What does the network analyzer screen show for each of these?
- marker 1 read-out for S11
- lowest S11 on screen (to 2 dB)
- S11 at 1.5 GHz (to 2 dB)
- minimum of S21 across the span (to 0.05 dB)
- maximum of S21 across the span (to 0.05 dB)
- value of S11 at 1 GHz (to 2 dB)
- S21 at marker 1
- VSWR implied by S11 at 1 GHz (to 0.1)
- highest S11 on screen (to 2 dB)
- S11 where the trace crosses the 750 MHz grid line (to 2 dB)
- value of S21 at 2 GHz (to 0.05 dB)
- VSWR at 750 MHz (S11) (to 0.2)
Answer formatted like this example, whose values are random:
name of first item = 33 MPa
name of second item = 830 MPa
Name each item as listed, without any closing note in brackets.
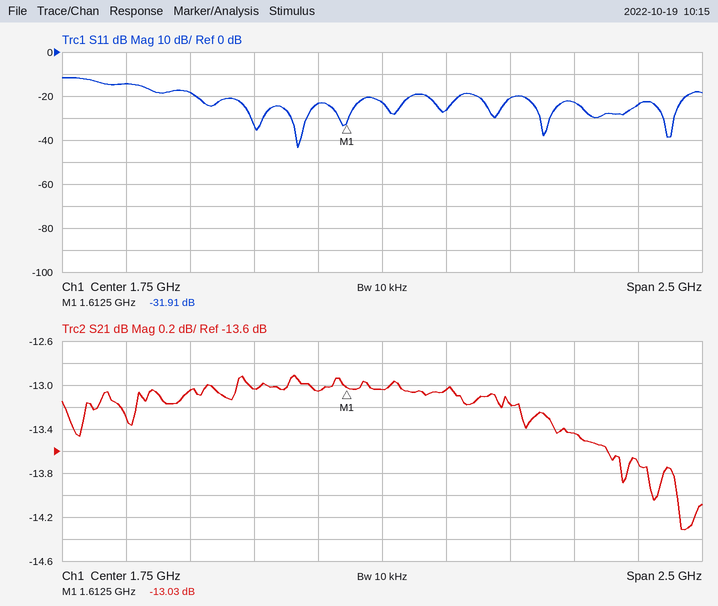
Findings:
marker 1 read-out for S11 = -31.91 dB
lowest S11 on screen = -44 dB
S11 at 1.5 GHz = -24 dB
minimum of S21 across the span = -14.30 dB
maximum of S21 across the span = -12.90 dB
value of S11 at 1 GHz = -18 dB
S21 at marker 1 = -13.03 dB
VSWR implied by S11 at 1 GHz = 1.3
highest S11 on screen = -12 dB
S11 where the trace crosses the 750 MHz grid line = -14 dB
value of S21 at 2 GHz = -13.05 dB
VSWR at 750 MHz (S11) = 1.4
